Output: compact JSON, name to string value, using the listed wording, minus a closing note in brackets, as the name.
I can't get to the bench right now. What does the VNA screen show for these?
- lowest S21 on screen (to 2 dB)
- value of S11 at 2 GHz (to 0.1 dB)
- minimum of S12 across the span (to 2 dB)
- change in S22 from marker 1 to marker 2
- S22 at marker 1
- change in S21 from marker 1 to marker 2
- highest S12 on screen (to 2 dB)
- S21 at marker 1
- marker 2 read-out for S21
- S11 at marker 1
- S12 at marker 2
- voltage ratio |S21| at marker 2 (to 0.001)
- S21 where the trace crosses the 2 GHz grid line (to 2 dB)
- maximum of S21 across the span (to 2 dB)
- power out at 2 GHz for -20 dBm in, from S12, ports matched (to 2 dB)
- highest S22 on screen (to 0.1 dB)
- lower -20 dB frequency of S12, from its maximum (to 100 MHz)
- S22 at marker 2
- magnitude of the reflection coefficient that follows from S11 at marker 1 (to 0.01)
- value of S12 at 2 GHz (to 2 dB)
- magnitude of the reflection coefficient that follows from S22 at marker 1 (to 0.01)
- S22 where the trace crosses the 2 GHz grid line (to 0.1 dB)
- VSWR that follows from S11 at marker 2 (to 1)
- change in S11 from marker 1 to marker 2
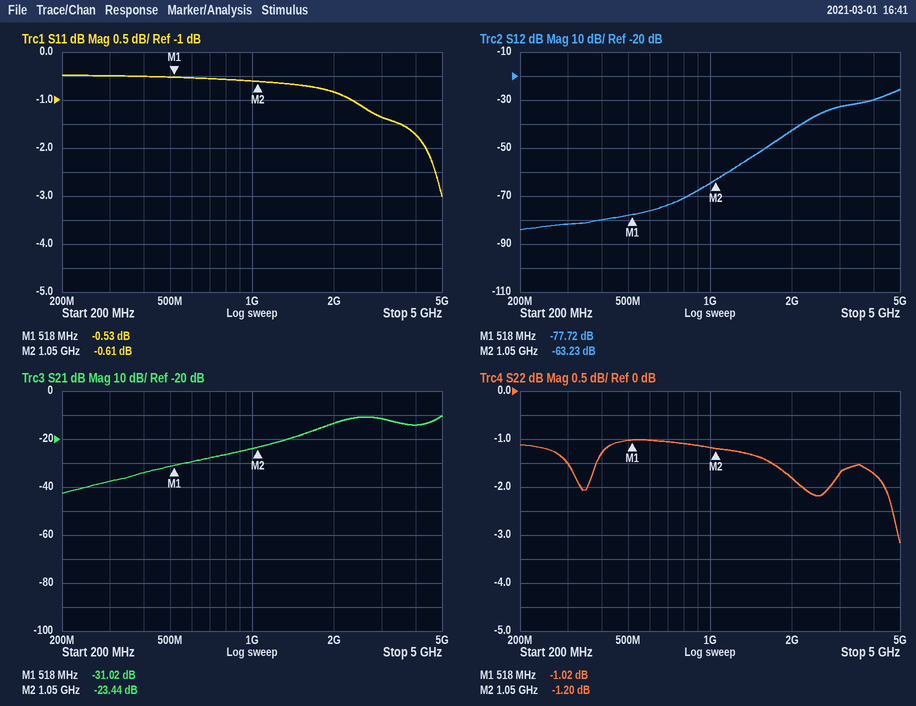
{"lowest S21 on screen": "-42 dB", "value of S11 at 2 GHz": "-0.8 dB", "minimum of S12 across the span": "-84 dB", "change in S22 from marker 1 to marker 2": "-0.18 dB", "S22 at marker 1": "-1.02 dB", "change in S21 from marker 1 to marker 2": "7.58 dB", "highest S12 on screen": "-26 dB", "S21 at marker 1": "-31.02 dB", "marker 2 read-out for S21": "-23.44 dB", "S11 at marker 1": "-0.53 dB", "S12 at marker 2": "-63.23 dB", "voltage ratio |S21| at marker 2": "0.067", "S21 where the trace crosses the 2 GHz grid line": "-14 dB", "maximum of S21 across the span": "-10 dB", "power out at 2 GHz for -20 dBm in, from S12, ports matched": "-62 dBm", "highest S22 on screen": "-1.0 dB", "lower -20 dB frequency of S12, from its maximum": "1.8 GHz", "S22 at marker 2": "-1.20 dB", "magnitude of the reflection coefficient that follows from S11 at marker 1": "0.94", "value of S12 at 2 GHz": "-42 dB", "magnitude of the reflection coefficient that follows from S22 at marker 1": "0.89", "S22 where the trace crosses the 2 GHz grid line": "-1.8 dB", "VSWR that follows from S11 at marker 2": "28", "change in S11 from marker 1 to marker 2": "-0.08 dB"}
